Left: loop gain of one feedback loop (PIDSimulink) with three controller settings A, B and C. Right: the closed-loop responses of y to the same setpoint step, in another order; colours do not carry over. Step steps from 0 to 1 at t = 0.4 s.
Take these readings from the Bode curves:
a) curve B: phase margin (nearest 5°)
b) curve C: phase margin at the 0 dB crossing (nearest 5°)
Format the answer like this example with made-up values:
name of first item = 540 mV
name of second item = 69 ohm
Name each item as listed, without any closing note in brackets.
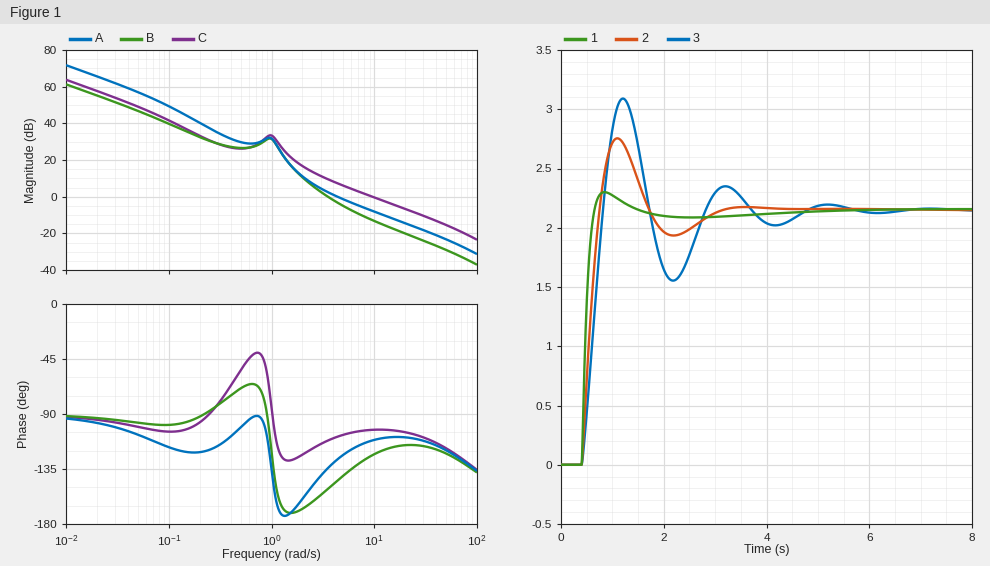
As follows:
curve B: phase margin = 30°
curve C: phase margin at the 0 dB crossing = 75°
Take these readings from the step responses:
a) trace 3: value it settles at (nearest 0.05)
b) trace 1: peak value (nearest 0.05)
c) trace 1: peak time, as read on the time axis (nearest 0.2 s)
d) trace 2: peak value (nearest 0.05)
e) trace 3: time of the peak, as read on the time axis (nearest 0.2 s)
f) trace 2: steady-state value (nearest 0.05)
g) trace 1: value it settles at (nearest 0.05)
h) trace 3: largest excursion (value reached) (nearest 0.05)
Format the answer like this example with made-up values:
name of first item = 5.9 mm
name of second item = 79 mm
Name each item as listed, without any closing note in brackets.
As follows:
trace 3: value it settles at = 2.15
trace 1: peak value = 2.30
trace 1: peak time, as read on the time axis = 0.8 s
trace 2: peak value = 2.75
trace 3: time of the peak, as read on the time axis = 1.2 s
trace 2: steady-state value = 2.15
trace 1: value it settles at = 2.15
trace 3: largest excursion (value reached) = 3.10
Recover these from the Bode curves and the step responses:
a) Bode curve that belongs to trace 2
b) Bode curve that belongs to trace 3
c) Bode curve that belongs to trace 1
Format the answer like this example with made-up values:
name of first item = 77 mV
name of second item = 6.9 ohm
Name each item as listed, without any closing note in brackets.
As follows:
Bode curve that belongs to trace 2 = A
Bode curve that belongs to trace 3 = B
Bode curve that belongs to trace 1 = C
